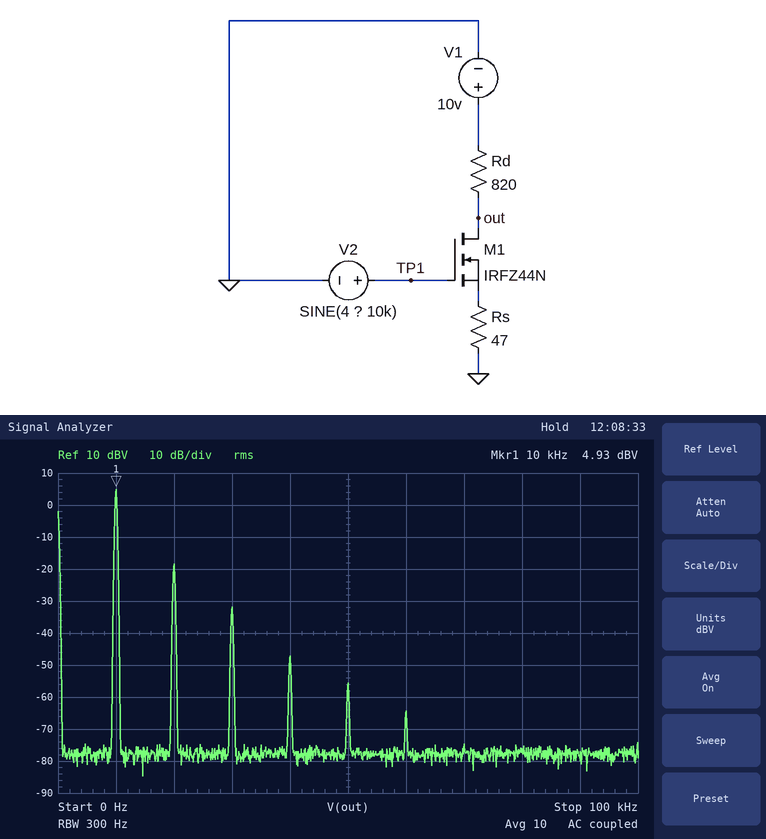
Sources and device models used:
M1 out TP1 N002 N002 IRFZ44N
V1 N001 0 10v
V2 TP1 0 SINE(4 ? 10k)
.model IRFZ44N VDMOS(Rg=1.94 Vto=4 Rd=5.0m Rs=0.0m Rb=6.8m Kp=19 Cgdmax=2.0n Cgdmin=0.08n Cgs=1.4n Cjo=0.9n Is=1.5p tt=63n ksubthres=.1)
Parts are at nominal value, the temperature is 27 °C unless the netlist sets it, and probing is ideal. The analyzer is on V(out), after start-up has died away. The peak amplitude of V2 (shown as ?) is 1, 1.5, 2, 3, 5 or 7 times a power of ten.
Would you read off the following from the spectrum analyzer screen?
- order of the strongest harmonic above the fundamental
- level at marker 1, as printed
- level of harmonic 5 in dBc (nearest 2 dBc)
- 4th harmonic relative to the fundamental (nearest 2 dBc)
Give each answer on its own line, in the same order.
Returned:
2
4.93 dBV
-60 dBc
-52 dBc
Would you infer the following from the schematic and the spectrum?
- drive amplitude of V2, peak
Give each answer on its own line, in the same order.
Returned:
200 mV
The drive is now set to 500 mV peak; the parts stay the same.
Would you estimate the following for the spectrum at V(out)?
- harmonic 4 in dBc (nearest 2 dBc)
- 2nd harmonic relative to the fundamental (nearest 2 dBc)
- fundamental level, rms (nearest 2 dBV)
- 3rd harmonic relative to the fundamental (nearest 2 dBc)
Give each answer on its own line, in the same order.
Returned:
-32 dBc
-14 dBc
12 dBV
-22 dBc
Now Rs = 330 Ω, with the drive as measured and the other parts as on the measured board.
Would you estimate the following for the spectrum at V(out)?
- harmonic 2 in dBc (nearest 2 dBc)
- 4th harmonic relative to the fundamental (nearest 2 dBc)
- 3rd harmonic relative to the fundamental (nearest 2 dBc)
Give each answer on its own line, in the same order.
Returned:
-30 dBc
-60 dBc
-44 dBc
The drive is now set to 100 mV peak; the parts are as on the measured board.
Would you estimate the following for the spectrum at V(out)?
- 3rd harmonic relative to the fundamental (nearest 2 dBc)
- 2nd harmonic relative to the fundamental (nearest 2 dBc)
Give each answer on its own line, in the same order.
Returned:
-50 dBc
-30 dBc
